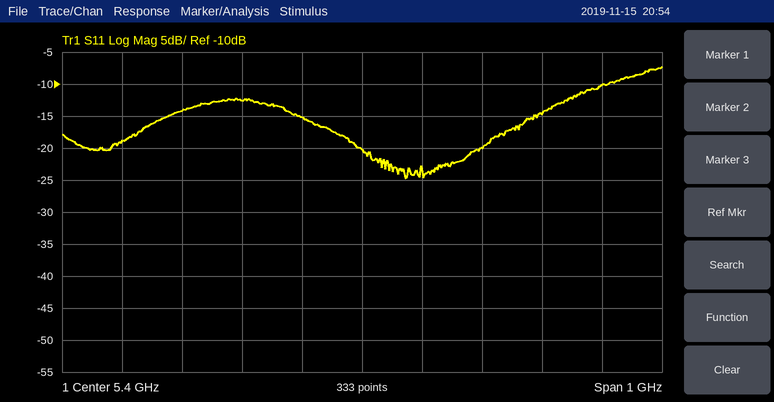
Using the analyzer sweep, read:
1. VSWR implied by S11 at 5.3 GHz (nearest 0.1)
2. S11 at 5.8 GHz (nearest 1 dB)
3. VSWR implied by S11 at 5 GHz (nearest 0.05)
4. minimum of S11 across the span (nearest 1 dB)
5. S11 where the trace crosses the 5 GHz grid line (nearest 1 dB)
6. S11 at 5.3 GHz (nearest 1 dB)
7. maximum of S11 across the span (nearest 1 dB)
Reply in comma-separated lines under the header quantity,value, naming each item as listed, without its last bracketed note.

quantity,value
VSWR implied by S11 at 5.3 GHz,1.4
S11 at 5.8 GHz,-10 dB
VSWR implied by S11 at 5 GHz,1.25
minimum of S11 across the span,-25 dB
S11 where the trace crosses the 5 GHz grid line,-19 dB
S11 at 5.3 GHz,-15 dB
maximum of S11 across the span,-7 dB
